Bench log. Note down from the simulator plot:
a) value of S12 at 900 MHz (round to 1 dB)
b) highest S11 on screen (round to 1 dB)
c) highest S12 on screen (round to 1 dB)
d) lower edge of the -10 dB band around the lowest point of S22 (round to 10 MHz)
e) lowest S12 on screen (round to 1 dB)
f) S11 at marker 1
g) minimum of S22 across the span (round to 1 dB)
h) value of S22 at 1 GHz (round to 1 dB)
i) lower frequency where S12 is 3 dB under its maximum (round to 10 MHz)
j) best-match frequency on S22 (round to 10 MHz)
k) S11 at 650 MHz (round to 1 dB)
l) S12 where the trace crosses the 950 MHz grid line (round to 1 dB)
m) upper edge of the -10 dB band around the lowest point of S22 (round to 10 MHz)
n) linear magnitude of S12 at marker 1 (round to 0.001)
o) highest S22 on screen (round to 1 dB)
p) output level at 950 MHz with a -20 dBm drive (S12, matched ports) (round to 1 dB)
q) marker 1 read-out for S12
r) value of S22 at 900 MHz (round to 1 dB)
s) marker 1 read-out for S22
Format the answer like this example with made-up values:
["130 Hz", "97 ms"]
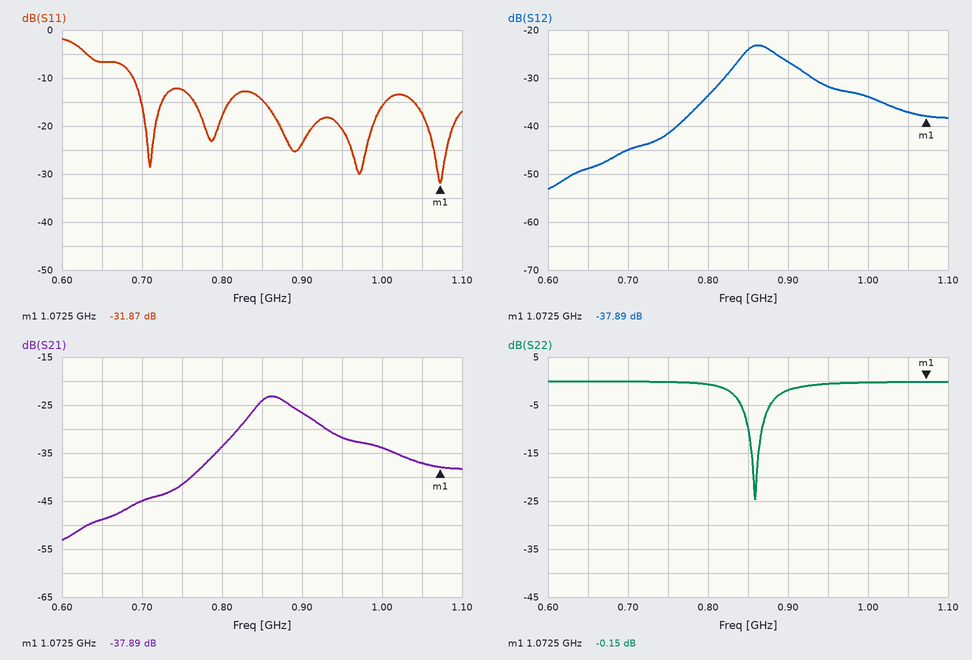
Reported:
["-27 dB", "-2 dB", "-23 dB", "850 MHz", "-53 dB", "-31.87 dB", "-25 dB", "0 dB", "840 MHz", "860 MHz", "-7 dB", "-32 dB", "870 MHz", "0.013", "0 dB", "-52 dBm", "-37.89 dB", "-2 dB", "-0.15 dB"]
